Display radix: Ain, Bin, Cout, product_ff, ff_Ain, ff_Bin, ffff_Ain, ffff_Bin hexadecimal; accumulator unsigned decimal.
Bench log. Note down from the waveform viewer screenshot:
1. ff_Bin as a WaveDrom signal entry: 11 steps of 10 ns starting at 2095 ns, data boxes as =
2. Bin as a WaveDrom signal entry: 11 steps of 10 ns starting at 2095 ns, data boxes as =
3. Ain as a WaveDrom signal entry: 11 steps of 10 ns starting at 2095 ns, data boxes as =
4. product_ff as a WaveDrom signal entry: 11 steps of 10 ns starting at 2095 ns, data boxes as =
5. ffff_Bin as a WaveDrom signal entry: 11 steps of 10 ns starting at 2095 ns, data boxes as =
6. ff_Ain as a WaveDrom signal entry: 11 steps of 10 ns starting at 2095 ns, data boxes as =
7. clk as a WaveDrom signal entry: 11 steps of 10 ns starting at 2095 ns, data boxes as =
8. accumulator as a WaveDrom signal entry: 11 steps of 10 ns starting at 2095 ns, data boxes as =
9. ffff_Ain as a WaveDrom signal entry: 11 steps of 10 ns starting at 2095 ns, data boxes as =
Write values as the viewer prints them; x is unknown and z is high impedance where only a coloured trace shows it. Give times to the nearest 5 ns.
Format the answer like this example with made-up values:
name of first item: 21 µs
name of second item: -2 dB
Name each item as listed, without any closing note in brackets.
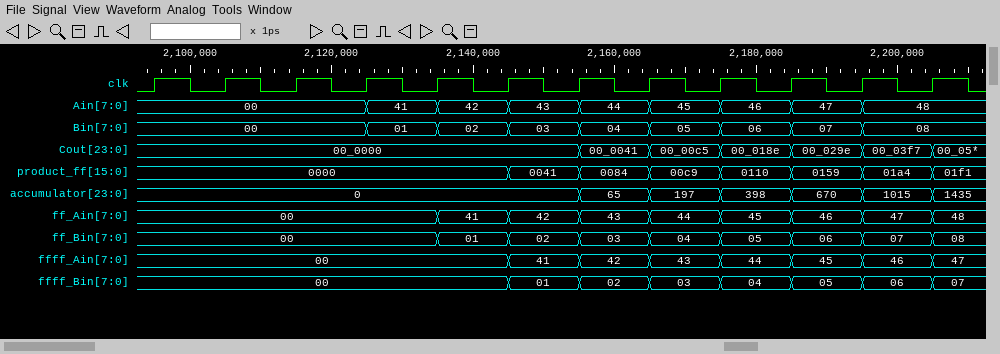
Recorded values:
ff_Bin as a WaveDrom signal entry: 11 steps of 10 ns starting at 2095 ns, data boxes as =: {name: 'ff_Bin', wave: '=...=======', data: '00 01 02 03 04 05 06 07'}
Bin as a WaveDrom signal entry: 11 steps of 10 ns starting at 2095 ns, data boxes as =: {name: 'Bin', wave: '=..========', data: '00 01 02 03 04 05 06 07 08'}
Ain as a WaveDrom signal entry: 11 steps of 10 ns starting at 2095 ns, data boxes as =: {name: 'Ain', wave: '=..========', data: '00 41 42 43 44 45 46 47 48'}
product_ff as a WaveDrom signal entry: 11 steps of 10 ns starting at 2095 ns, data boxes as =: {name: 'product_ff', wave: '=....======', data: '0000 0041 0084 00c9 0110 0159 01a4'}
ffff_Bin as a WaveDrom signal entry: 11 steps of 10 ns starting at 2095 ns, data boxes as =: {name: 'ffff_Bin', wave: '=....======', data: '00 01 02 03 04 05 06'}
ff_Ain as a WaveDrom signal entry: 11 steps of 10 ns starting at 2095 ns, data boxes as =: {name: 'ff_Ain', wave: '=...=======', data: '00 41 42 43 44 45 46 47'}
clk as a WaveDrom signal entry: 11 steps of 10 ns starting at 2095 ns, data boxes as =: {name: 'clk', wave: 'p..........'}
accumulator as a WaveDrom signal entry: 11 steps of 10 ns starting at 2095 ns, data boxes as =: {name: 'accumulator', wave: '=.....=====', data: '0 65 197 398 670 1015'}
ffff_Ain as a WaveDrom signal entry: 11 steps of 10 ns starting at 2095 ns, data boxes as =: {name: 'ffff_Ain', wave: '=....======', data: '00 41 42 43 44 45 46'}
